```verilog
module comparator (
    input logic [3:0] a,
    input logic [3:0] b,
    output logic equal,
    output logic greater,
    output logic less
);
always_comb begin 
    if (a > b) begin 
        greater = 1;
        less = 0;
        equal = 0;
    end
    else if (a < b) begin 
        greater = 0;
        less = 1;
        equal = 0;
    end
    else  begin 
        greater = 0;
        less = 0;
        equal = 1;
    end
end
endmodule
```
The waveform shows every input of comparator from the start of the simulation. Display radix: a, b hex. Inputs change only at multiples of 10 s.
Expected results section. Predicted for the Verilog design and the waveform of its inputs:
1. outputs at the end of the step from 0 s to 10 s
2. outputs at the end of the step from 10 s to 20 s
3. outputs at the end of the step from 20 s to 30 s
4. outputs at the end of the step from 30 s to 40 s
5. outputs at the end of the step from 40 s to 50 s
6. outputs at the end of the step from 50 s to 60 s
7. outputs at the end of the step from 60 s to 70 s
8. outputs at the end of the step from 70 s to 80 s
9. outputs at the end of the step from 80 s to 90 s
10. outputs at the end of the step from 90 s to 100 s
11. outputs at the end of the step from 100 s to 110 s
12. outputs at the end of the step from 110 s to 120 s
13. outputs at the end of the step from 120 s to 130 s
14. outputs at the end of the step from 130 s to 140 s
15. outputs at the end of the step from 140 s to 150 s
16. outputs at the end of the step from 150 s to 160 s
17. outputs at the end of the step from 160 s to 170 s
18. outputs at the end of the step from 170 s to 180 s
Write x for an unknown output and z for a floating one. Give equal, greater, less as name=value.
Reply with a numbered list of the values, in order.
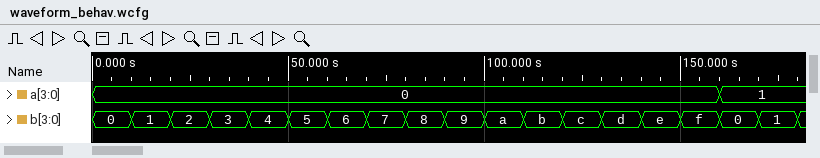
1. equal=1, greater=0, less=0
2. equal=0, greater=0, less=1
3. equal=0, greater=0, less=1
4. equal=0, greater=0, less=1
5. equal=0, greater=0, less=1
6. equal=0, greater=0, less=1
7. equal=0, greater=0, less=1
8. equal=0, greater=0, less=1
9. equal=0, greater=0, less=1
10. equal=0, greater=0, less=1
11. equal=0, greater=0, less=1
12. equal=0, greater=0, less=1
13. equal=0, greater=0, less=1
14. equal=0, greater=0, less=1
15. equal=0, greater=0, less=1
16. equal=0, greater=0, less=1
17. equal=0, greater=1, less=0
18. equal=1, greater=0, less=0
